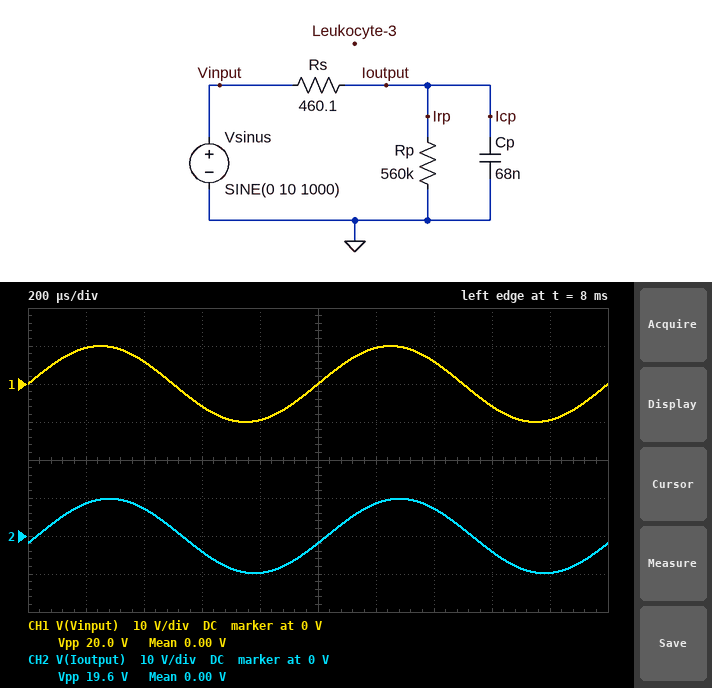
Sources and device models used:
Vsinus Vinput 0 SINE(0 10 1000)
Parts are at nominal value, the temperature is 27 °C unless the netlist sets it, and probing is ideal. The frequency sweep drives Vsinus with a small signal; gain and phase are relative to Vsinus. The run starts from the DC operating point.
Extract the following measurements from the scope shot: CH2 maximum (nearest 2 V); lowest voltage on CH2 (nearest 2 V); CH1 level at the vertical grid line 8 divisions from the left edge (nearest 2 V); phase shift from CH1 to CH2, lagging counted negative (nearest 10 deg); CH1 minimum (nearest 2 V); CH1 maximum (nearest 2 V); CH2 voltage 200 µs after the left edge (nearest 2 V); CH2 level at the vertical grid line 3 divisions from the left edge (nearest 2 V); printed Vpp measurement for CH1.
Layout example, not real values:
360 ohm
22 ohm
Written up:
10 V
-10 V
-6 V
-10 deg
-10 V
10 V
8 V
-4 V
20.0 V
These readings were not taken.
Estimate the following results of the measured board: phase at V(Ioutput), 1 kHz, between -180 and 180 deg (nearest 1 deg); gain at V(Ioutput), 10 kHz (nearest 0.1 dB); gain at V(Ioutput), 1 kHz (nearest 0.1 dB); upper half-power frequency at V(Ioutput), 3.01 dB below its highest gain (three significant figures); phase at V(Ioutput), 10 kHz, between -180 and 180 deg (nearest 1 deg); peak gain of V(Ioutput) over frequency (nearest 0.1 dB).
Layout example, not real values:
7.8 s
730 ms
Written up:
-11 deg
-6.9 dB
-0.2 dB
5.09 kHz
-63 deg
0 dB
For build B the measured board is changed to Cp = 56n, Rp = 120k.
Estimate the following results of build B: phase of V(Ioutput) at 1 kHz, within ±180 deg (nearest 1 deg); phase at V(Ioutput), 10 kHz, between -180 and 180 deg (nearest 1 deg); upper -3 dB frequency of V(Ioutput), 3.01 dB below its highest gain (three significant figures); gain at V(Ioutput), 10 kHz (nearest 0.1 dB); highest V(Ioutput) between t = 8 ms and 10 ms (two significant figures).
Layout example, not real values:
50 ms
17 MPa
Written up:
-9 deg
-58 deg
6.20 kHz
-5.6 dB
9.8 V
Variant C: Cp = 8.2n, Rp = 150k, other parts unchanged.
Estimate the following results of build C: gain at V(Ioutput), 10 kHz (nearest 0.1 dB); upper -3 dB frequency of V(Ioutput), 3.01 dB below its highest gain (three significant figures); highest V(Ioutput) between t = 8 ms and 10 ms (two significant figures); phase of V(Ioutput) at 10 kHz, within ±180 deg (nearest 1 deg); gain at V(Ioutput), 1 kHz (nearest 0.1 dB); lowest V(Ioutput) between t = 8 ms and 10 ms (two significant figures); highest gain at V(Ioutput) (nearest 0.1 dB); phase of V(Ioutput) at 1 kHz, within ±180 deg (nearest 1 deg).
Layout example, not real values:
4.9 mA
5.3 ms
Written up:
-0.3 dB
42.3 kHz
10 V
-13 deg
0 dB
-10 V
0 dB
-1 deg
